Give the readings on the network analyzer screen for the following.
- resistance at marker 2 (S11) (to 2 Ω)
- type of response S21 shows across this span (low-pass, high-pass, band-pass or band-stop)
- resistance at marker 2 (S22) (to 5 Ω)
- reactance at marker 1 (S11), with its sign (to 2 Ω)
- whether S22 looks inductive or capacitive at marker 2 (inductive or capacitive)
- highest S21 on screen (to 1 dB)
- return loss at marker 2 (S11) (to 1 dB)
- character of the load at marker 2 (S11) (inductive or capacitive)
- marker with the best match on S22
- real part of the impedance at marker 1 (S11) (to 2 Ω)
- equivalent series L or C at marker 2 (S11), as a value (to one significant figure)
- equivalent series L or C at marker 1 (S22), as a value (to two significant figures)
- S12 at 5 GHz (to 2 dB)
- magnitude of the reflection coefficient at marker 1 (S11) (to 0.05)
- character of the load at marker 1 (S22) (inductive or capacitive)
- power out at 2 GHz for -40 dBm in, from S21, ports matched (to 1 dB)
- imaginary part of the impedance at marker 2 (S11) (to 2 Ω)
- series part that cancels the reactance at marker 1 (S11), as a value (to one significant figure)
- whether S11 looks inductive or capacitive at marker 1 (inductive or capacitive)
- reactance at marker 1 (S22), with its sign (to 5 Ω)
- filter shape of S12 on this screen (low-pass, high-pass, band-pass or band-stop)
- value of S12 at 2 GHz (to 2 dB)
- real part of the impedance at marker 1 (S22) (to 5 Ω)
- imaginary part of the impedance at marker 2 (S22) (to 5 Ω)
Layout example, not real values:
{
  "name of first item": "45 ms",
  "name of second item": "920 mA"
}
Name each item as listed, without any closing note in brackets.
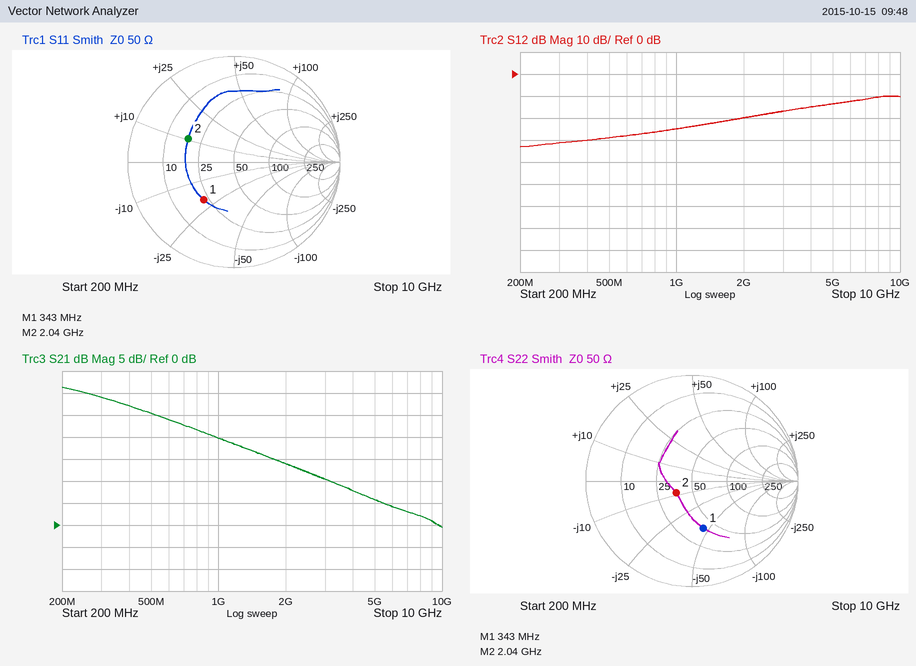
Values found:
{
  "resistance at marker 2 (S11)": "18 Ω",
  "type of response S21 shows across this span": "low-pass",
  "resistance at marker 2 (S22)": "35 Ω",
  "reactance at marker 1 (S11), with its sign": "-20 Ω",
  "whether S22 looks inductive or capacitive at marker 2": "capacitive",
  "highest S21 on screen": "31 dB",
  "return loss at marker 2 (S11)": "6 dB",
  "character of the load at marker 2 (S11)": "inductive",
  "marker with the best match on S22": "marker 2",
  "real part of the impedance at marker 1 (S11)": "22 Ω",
  "equivalent series L or C at marker 2 (S11), as a value": "800 pH",
  "equivalent series L or C at marker 1 (S22), as a value": "10 pF",
  "S12 at 5 GHz": "-14 dB",
  "magnitude of the reflection coefficient at marker 1 (S11)": "0.45",
  "character of the load at marker 1 (S22)": "capacitive",
  "power out at 2 GHz for -40 dBm in, from S21, ports matched": "-26 dBm",
  "imaginary part of the impedance at marker 2 (S11)": "+10 Ω",
  "series part that cancels the reactance at marker 1 (S11), as a value": "9 nH",
  "whether S11 looks inductive or capacitive at marker 1": "capacitive",
  "reactance at marker 1 (S22), with its sign": "-45 Ω",
  "filter shape of S12 on this screen": "high-pass",
  "value of S12 at 2 GHz": "-20 dB",
  "real part of the impedance at marker 1 (S22)": "40 Ω",
  "imaginary part of the impedance at marker 2 (S22)": "-10 Ω"
}
